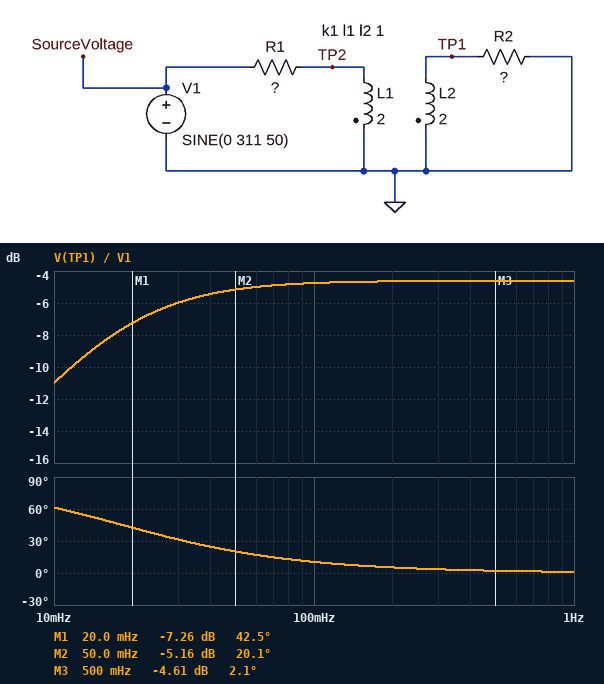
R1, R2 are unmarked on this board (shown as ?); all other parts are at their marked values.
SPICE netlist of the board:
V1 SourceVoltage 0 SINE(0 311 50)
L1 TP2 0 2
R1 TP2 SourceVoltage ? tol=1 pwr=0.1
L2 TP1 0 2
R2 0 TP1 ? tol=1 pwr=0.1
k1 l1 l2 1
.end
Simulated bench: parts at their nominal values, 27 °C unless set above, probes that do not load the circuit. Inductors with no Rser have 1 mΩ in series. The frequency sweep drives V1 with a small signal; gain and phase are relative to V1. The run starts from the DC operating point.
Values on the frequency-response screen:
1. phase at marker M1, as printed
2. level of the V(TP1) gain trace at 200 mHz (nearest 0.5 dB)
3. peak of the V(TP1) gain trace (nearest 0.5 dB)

42.5 deg
-4.5 dB
-4.5 dB
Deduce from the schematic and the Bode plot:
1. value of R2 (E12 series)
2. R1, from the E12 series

0.56 Ω
0.39 Ω
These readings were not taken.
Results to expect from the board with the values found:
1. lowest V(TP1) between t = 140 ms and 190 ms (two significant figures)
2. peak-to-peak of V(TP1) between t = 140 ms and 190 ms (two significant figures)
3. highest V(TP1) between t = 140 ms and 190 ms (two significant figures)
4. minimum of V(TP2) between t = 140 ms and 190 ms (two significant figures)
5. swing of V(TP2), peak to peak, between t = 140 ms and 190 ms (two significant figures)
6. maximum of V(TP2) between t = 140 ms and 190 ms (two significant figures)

-180 V
370 V
180 V
-180 V
370 V
180 V
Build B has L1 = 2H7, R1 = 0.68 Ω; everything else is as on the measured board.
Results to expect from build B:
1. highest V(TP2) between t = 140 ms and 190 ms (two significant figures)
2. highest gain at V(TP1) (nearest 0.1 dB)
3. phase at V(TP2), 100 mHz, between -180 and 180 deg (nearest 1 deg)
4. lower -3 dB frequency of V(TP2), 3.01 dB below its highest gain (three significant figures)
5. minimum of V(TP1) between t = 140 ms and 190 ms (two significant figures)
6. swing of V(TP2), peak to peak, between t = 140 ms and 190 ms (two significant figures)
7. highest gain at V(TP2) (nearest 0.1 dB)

160 V
-6.9 dB
12 deg
21.1 mHz
-140 V
330 V
-5.6 dB
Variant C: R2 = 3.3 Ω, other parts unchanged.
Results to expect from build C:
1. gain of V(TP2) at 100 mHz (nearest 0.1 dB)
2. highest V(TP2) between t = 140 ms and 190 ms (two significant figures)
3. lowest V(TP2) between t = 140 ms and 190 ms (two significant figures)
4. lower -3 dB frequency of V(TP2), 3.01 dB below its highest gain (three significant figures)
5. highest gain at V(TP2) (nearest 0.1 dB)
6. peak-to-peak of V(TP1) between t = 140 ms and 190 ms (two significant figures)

-1.3 dB
280 V
-280 V
27.8 mHz
-1.0 dB
560 V
